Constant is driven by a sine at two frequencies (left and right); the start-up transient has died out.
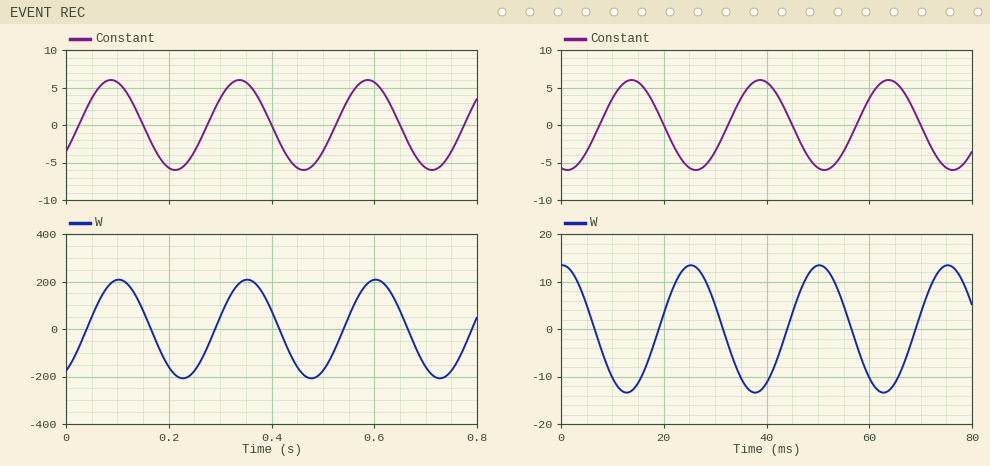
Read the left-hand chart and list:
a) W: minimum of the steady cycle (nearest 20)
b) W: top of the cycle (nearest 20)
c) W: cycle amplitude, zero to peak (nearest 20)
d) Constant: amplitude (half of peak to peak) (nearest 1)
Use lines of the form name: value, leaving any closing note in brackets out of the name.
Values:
W: minimum of the steady cycle: -200
W: top of the cycle: 200
W: cycle amplitude, zero to peak: 200
Constant: amplitude (half of peak to peak): 6
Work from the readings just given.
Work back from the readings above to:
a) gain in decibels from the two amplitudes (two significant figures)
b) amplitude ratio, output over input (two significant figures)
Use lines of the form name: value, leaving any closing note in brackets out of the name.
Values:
gain in decibels from the two amplitudes: 30 dB
amplitude ratio, output over input: 33
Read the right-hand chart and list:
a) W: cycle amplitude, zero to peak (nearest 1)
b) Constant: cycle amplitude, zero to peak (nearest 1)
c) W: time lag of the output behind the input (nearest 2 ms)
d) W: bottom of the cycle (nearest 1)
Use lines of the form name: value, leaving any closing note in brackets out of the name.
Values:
W: cycle amplitude, zero to peak: 13
Constant: cycle amplitude, zero to peak: 6
W: time lag of the output behind the input: 12 ms
W: bottom of the cycle: -13
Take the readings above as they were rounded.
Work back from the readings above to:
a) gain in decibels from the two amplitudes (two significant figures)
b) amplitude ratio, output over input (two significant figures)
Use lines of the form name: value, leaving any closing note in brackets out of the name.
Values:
gain in decibels from the two amplitudes: 6.7 dB
amplitude ratio, output over input: 2.2
